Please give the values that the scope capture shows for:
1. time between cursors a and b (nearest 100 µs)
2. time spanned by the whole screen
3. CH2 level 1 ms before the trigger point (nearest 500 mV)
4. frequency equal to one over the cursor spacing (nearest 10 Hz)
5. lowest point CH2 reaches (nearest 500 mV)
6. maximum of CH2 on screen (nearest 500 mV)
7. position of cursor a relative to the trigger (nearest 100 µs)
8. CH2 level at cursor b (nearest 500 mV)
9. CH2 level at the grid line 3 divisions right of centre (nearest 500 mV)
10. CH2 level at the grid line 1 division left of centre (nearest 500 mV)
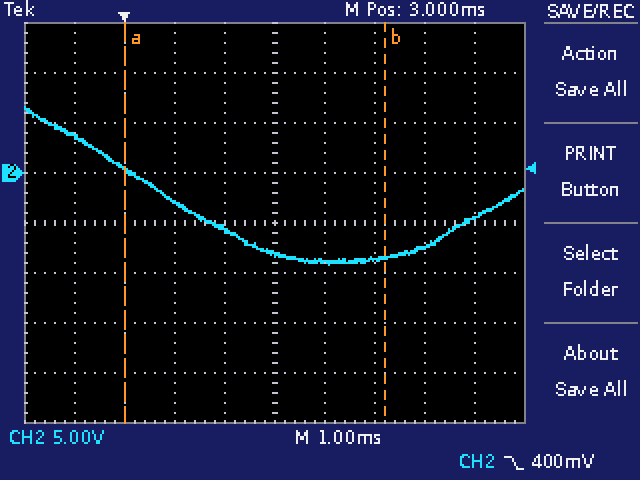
5.2 ms
10 ms
3.5 V
190 Hz
-9.0 V
6.5 V
0.0 ms
-8.5 V
-7.5 V
-5.5 V
